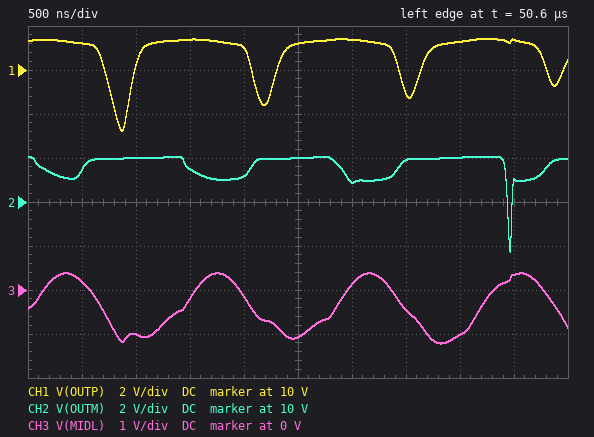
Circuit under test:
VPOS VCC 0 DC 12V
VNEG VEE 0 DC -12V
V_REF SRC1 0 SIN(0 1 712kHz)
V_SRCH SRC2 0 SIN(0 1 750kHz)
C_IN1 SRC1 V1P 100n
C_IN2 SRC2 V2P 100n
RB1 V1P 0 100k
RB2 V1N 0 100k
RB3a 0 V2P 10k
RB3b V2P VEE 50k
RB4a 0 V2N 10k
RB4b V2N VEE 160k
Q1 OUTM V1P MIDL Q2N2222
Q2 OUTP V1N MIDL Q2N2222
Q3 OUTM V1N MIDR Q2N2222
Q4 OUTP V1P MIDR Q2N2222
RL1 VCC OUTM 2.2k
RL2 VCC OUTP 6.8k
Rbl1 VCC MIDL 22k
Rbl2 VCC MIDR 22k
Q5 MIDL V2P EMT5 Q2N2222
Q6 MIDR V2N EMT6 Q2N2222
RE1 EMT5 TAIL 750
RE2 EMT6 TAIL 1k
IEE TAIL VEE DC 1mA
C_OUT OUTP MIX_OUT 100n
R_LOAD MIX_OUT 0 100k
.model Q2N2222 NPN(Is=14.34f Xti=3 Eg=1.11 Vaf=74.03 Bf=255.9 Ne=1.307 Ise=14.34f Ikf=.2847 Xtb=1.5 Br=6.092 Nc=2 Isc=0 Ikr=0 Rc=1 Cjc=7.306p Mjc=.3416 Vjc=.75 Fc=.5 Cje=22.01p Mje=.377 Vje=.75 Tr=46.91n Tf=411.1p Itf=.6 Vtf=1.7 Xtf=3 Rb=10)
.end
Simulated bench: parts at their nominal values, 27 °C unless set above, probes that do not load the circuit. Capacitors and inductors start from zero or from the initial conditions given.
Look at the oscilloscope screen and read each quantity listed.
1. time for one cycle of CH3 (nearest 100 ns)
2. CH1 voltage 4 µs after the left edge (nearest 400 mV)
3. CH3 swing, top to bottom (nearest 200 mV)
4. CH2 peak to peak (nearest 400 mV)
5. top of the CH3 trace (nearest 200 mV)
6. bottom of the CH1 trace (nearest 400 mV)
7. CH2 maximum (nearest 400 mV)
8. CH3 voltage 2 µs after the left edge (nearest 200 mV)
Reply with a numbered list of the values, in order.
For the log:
1. 1.4 µs
2. 11.2 V
3. 1.6 V
4. 4.4 V
5. 400 mV
6. 7.2 V
7. 12.0 V
8. -200 mV
